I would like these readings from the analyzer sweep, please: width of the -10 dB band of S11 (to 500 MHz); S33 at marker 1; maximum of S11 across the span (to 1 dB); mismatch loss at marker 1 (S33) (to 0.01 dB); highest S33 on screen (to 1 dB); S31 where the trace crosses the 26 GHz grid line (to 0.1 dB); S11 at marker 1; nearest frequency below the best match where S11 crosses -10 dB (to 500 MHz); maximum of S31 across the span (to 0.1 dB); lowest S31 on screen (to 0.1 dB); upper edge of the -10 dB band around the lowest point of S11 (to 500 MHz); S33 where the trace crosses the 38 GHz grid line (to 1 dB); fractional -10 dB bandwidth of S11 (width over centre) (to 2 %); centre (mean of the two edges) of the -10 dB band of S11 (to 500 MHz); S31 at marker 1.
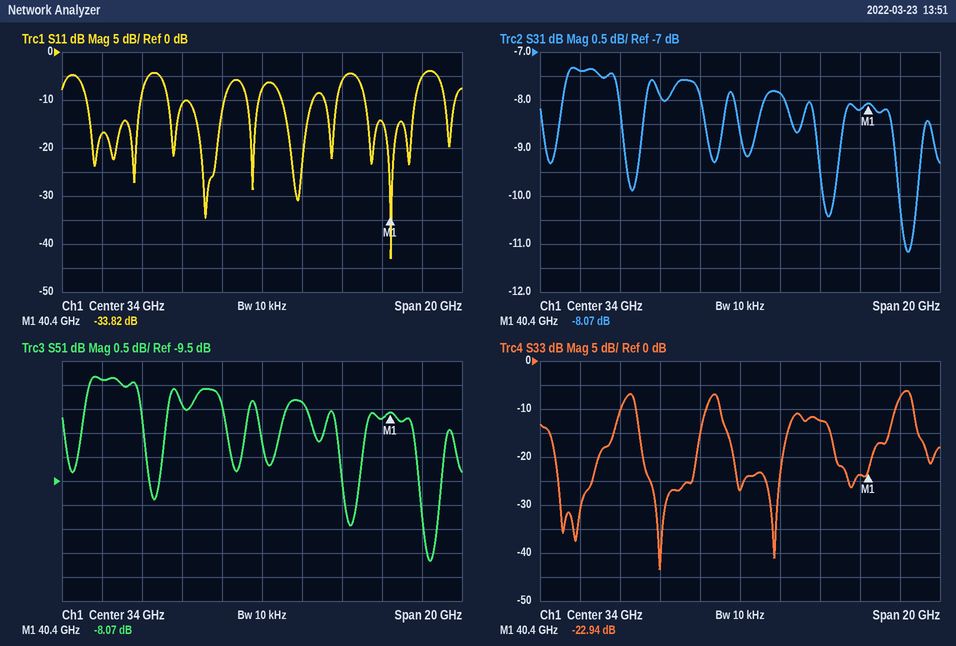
2.5 GHz
-22.94 dB
-4 dB
0.02 dB
-6 dB
-7.4 dB
-33.82 dB
39.0 GHz
-7.3 dB
-11.2 dB
41.5 GHz
-12 dB
6 %
40.5 GHz
-8.07 dB
